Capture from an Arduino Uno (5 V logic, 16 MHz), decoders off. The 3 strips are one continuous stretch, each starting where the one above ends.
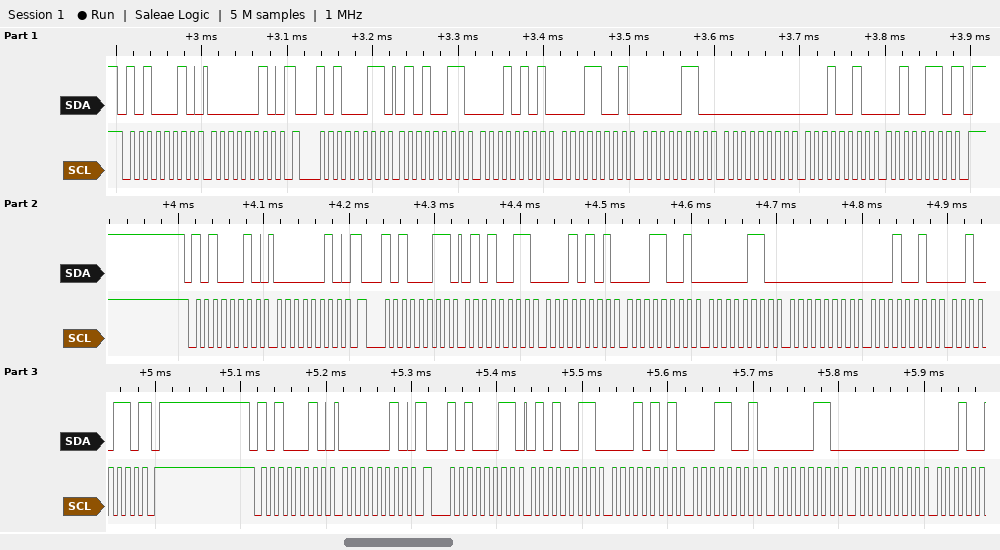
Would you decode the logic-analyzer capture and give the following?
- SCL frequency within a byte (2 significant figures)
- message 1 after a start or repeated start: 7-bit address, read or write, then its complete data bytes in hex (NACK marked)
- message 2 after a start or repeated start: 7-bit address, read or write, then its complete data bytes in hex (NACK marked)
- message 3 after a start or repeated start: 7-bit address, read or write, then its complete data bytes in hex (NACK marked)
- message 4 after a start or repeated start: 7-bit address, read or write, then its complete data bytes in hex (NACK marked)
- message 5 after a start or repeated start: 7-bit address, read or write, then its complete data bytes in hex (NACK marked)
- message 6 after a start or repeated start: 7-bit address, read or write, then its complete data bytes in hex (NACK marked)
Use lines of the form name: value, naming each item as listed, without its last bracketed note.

SCL frequency within a byte: 100 kHz
message 1 after a start or repeated start: 7-bit address, read or write, then its complete data bytes in hex: 0x51 write: 02
message 2 after a start or repeated start: 7-bit address, read or write, then its complete data bytes in hex: 0x51 read: 53 15 19 06 00 12 26 NACK
message 3 after a start or repeated start: 7-bit address, read or write, then its complete data bytes in hex: 0x51 write: 02
message 4 after a start or repeated start: 7-bit address, read or write, then its complete data bytes in hex: 0x51 read: 53 15 19 06 00 12 26 NACK
message 5 after a start or repeated start: 7-bit address, read or write, then its complete data bytes in hex: 0x51 write: 02
message 6 after a start or repeated start: 7-bit address, read or write, then its complete data bytes in hex: 0x51 read: 53 15 19 06 00
